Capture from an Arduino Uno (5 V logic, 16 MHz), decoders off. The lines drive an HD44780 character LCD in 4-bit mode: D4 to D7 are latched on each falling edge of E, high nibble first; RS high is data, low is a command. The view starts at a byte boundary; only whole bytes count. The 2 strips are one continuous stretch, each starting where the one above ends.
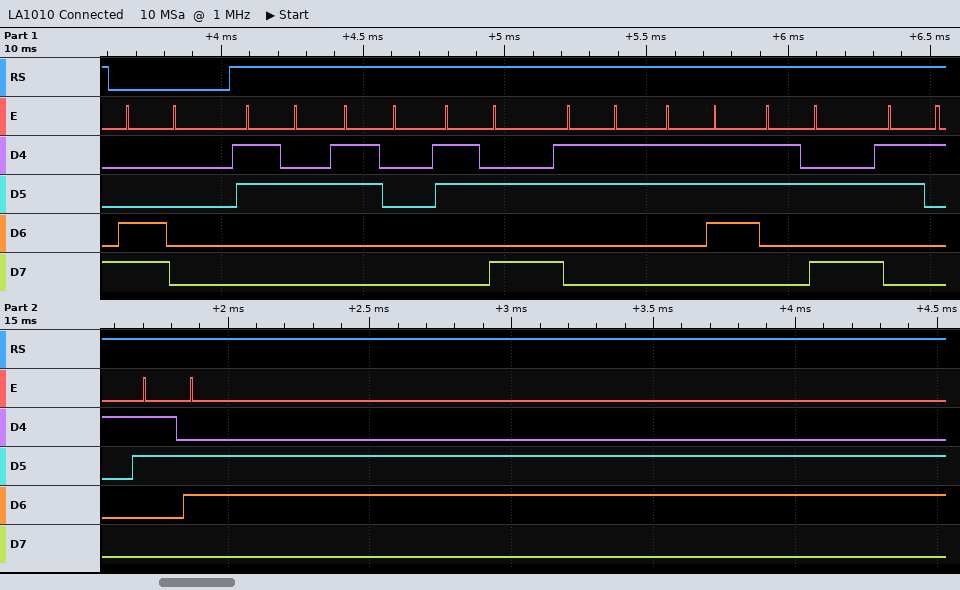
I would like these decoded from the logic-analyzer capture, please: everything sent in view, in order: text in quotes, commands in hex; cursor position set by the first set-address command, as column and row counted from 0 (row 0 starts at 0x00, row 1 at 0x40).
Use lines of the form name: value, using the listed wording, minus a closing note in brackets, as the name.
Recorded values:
everything sent in view, in order: text in quotes, commands in hex: 0xC0 "20:37:16"
cursor position set by the first set-address command, as column and row counted from 0: column 0, row 1
